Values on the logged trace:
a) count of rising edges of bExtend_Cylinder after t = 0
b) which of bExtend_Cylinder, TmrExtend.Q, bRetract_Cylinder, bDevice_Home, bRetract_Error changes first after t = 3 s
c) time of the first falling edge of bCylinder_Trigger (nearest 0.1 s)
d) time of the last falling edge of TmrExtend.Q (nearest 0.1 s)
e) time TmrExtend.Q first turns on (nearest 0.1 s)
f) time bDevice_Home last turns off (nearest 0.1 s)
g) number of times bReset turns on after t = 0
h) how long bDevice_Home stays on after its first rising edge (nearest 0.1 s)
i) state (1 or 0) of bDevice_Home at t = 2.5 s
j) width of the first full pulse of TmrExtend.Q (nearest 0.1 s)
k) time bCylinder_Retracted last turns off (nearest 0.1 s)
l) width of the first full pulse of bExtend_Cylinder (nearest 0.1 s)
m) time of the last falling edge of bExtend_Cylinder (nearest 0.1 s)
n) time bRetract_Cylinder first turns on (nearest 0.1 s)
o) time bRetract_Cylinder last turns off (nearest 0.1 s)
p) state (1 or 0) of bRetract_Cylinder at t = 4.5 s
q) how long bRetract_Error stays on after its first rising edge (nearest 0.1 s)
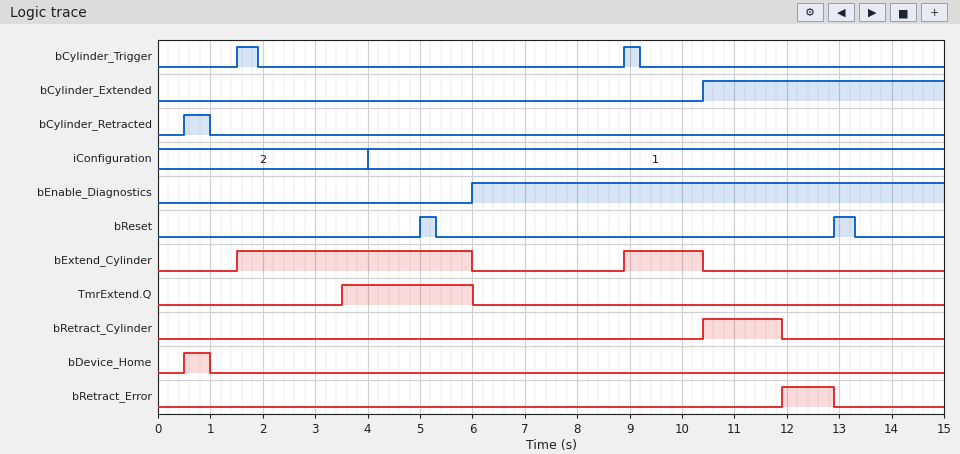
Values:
2
TmrExtend.Q
1.9 s
6.0 s
3.5 s
1.0 s
2
0.5 s
0
2.5 s
1.0 s
4.5 s
10.4 s
10.4 s
11.9 s
0
1.0 s
